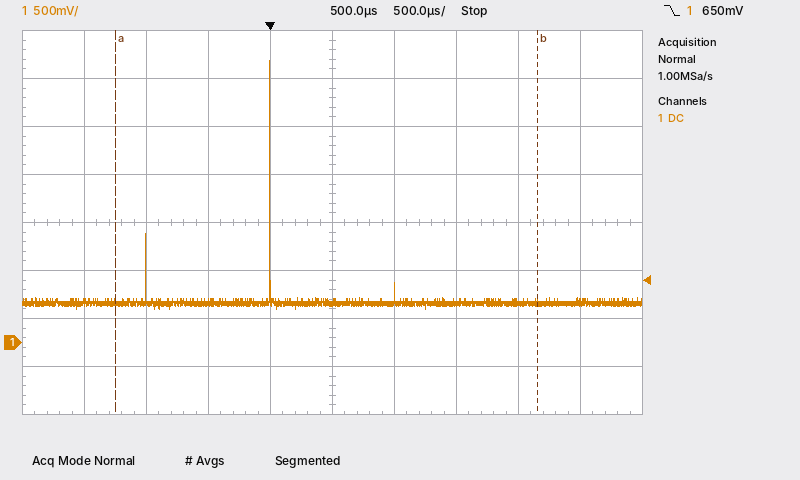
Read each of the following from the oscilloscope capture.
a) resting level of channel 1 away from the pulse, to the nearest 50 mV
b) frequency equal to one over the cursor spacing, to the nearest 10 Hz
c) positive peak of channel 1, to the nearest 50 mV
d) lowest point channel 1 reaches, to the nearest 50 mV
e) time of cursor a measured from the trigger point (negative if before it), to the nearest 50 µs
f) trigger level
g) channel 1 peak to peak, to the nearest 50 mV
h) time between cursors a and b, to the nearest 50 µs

400 mV
290 Hz
2.95 V
350 mV
-1.25 ms
650 mV
2.60 V
3.40 ms
